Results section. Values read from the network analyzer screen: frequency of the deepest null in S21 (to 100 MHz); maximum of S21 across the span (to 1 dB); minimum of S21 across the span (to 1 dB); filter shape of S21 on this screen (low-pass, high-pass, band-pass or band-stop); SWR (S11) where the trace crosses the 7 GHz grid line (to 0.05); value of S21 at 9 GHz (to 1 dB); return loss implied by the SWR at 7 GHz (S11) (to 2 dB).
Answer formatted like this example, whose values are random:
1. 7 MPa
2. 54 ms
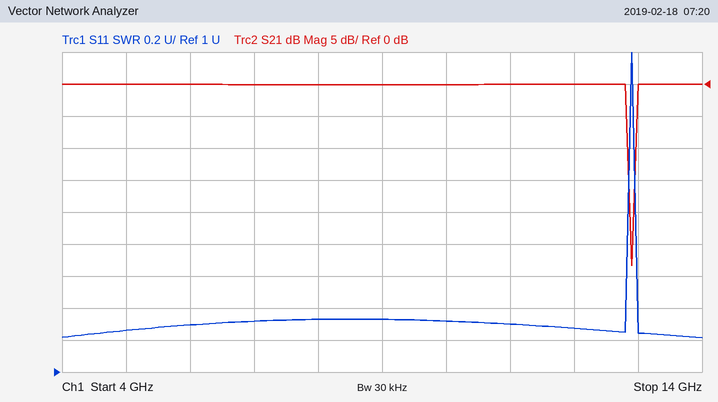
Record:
1. 12.9 GHz
2. 0 dB
3. -28 dB
4. band-stop
5. 1.30
6. 0 dB
7. 18 dB
